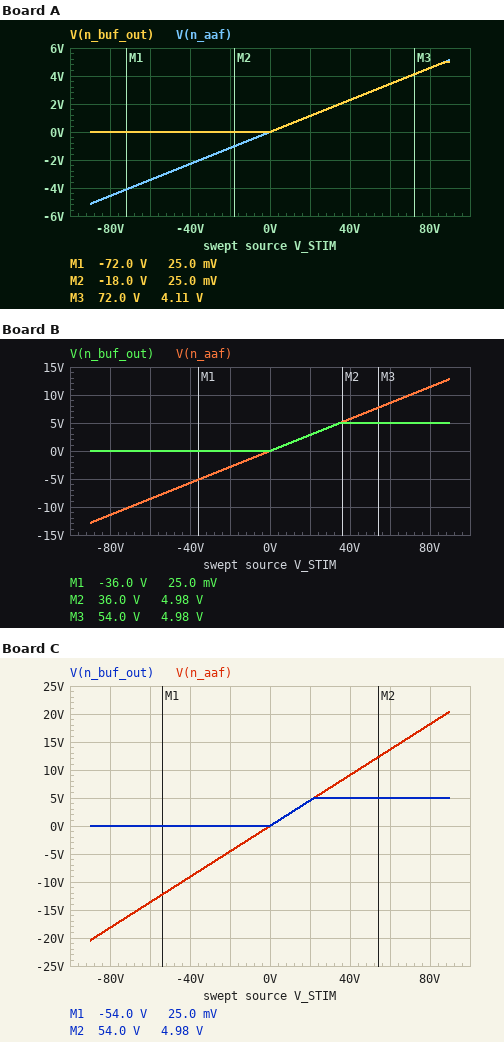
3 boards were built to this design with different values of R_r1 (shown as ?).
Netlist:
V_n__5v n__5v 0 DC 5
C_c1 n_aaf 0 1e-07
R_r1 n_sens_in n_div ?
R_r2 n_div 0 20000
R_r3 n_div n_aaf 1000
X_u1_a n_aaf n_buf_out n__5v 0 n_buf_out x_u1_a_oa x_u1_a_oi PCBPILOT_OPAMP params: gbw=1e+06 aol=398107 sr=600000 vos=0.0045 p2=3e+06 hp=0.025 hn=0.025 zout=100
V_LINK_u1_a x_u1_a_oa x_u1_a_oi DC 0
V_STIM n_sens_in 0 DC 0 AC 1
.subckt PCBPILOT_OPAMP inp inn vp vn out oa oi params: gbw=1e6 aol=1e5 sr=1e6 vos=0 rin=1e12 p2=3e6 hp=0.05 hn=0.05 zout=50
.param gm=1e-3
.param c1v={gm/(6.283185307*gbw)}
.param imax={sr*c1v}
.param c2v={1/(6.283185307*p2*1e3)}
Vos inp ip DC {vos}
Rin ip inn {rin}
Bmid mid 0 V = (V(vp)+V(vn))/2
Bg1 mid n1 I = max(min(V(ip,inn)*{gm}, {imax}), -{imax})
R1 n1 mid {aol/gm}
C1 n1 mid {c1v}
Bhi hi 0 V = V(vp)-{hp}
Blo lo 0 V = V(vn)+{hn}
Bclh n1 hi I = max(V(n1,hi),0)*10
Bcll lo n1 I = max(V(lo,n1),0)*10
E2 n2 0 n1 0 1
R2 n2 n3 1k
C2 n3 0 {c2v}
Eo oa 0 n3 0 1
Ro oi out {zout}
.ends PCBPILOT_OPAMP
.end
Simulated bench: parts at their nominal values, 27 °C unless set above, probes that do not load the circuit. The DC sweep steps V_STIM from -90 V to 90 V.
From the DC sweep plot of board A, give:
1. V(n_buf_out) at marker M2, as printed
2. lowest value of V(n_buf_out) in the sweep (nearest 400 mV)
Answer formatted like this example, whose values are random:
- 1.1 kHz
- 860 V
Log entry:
- 25.0 mV
- 0 V
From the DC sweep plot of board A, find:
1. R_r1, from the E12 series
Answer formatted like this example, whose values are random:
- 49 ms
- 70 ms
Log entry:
- 330 kΩ
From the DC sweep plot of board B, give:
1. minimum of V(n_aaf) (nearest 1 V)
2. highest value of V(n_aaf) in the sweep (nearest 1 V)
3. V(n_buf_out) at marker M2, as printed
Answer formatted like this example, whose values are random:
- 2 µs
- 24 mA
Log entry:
- -13 V
- 13 V
- 4.98 V
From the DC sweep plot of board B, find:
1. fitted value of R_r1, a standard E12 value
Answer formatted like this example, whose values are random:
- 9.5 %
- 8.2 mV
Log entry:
- 120 kΩ
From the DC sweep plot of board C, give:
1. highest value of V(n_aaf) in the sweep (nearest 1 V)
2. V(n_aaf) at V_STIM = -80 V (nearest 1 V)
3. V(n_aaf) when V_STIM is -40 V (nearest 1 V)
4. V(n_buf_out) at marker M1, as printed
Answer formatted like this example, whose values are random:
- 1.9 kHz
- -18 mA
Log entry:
- 20 V
- -18 V
- -9 V
- 25.0 mV
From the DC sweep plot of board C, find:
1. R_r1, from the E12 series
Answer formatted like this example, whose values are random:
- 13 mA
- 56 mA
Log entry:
- 68 kΩ
